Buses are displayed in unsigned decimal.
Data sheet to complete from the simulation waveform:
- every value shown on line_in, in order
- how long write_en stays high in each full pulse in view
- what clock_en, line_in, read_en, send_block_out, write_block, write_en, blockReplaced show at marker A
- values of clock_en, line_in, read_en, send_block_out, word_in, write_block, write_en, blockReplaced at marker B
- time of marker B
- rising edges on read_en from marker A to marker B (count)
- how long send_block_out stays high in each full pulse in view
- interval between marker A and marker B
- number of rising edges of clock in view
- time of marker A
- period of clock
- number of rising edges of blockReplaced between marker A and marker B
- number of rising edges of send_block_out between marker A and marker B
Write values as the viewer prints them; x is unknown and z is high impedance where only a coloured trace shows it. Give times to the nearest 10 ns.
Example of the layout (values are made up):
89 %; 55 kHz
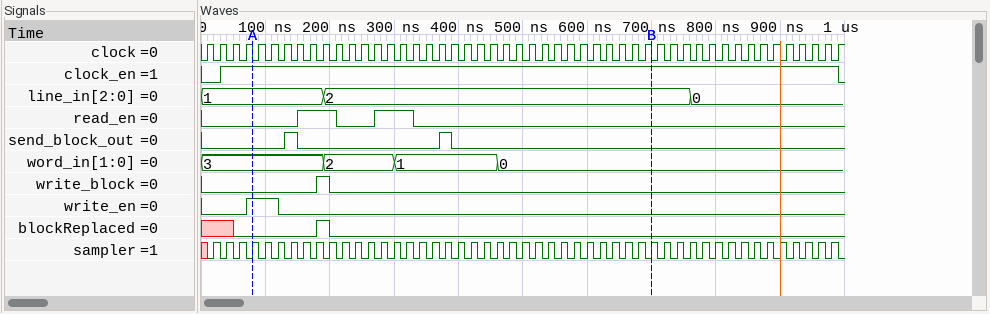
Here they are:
1, 2, 0; 50 ns; clock_en=1, line_in=1, read_en=0, send_block_out=0, write_block=0, write_en=1, blockReplaced=0; clock_en=1, line_in=2, read_en=0, send_block_out=0, word_in=0, write_block=0, write_en=0, blockReplaced=0; 700 ns; 2; 20 ns, 20 ns; 620 ns; 50; 80 ns; 20 ns; 1; 2
